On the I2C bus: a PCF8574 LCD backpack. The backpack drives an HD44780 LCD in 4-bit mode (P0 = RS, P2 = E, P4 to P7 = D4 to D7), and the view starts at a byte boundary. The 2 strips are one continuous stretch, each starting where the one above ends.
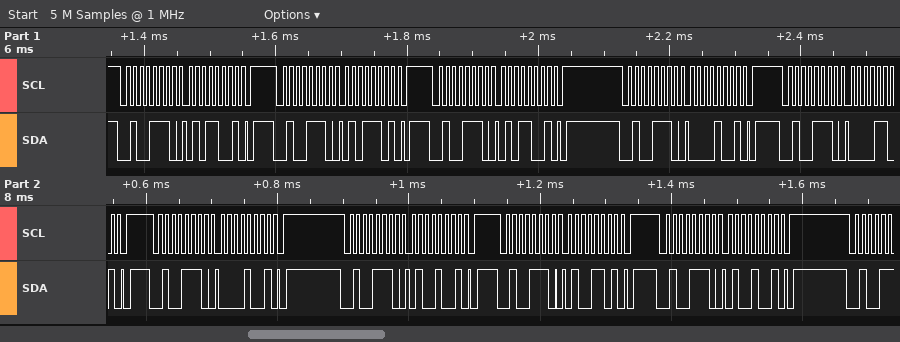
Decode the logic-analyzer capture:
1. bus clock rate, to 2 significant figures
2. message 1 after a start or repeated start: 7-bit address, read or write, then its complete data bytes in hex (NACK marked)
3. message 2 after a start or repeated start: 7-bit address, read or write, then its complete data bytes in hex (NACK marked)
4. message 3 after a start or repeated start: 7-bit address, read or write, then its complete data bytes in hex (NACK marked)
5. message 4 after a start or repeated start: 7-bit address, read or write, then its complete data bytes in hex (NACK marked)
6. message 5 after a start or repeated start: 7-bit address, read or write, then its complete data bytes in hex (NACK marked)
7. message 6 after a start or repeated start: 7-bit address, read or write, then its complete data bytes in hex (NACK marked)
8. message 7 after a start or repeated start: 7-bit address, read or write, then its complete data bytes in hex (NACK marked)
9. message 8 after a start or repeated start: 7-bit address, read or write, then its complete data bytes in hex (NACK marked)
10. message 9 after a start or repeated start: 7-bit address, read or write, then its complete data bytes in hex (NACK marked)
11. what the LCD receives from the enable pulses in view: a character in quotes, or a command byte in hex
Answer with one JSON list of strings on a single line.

["100 kHz", "0x27 write: 59", "0x27 write: 5D", "0x27 write: 59", "0x27 write: 09", "0x27 write: 0D", "0x27 write: 09", "0x27 write: 49", "0x27 write: 4D", "0x27 write: 49", "'P'"]
